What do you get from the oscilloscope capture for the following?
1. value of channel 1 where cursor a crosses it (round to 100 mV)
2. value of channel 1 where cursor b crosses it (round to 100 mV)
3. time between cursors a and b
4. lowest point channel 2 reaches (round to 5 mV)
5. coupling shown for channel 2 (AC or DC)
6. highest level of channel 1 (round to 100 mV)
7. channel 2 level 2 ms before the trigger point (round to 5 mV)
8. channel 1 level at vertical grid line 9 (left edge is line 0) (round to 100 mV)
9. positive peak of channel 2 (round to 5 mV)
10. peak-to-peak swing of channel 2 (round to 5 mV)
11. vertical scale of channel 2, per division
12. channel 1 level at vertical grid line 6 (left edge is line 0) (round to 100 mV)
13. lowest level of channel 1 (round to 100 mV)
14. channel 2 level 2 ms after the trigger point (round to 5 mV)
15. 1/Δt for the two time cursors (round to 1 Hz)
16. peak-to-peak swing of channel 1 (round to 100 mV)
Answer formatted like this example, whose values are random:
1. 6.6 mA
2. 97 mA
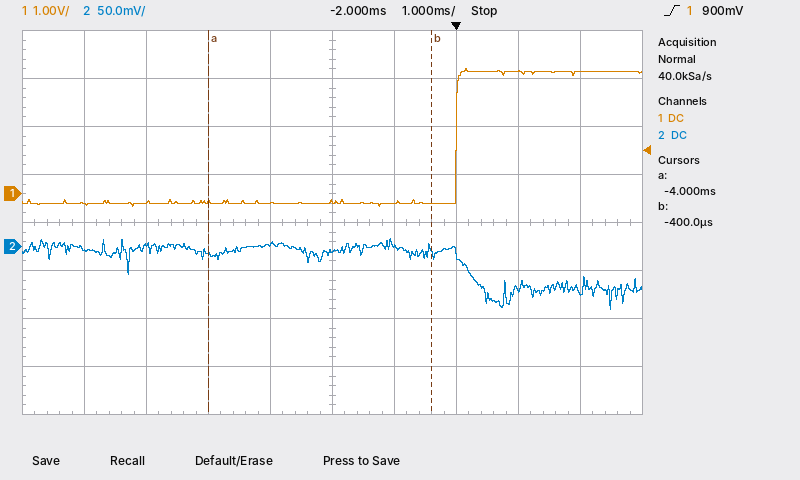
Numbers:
1. -200 mV
2. -200 mV
3. 3.6 ms
4. -65 mV
5. DC
6. 2.6 V
7. -5 mV
8. 2.5 V
9. 10 mV
10. 75 mV
11. 50 mV
12. -200 mV
13. -300 mV
14. -45 mV
15. 278 Hz
16. 2.9 V
